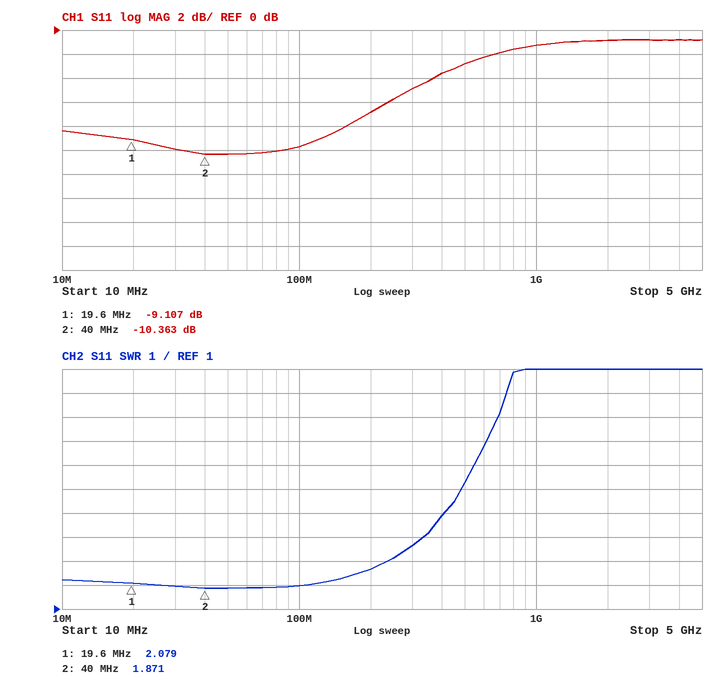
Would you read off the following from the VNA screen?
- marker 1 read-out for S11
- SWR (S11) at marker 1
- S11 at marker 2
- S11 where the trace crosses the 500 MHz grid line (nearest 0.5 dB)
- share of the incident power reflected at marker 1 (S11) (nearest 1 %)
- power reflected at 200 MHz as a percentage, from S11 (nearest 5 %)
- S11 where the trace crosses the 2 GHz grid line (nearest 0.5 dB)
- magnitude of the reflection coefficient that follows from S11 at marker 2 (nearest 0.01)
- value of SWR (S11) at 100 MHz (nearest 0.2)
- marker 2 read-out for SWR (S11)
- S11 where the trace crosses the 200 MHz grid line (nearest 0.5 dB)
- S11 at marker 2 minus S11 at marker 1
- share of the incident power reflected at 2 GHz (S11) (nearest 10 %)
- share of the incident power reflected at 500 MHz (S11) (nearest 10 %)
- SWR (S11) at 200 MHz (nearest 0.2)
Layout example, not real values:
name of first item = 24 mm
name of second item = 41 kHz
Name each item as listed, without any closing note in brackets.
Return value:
marker 1 read-out for S11 = -9.107 dB
SWR (S11) at marker 1 = 2.079
S11 at marker 2 = -10.363 dB
S11 where the trace crosses the 500 MHz grid line = -3.0 dB
share of the incident power reflected at marker 1 (S11) = 12 %
power reflected at 200 MHz as a percentage, from S11 = 20 %
S11 where the trace crosses the 2 GHz grid line = -1.0 dB
magnitude of the reflection coefficient that follows from S11 at marker 2 = 0.30
value of SWR (S11) at 100 MHz = 2.0
marker 2 read-out for SWR = 1.871
S11 where the trace crosses the 200 MHz grid line = -7.0 dB
S11 at marker 2 minus S11 at marker 1 = -1.256 dB
share of the incident power reflected at 2 GHz (S11) = 80 %
share of the incident power reflected at 500 MHz (S11) = 50 %
SWR (S11) at 200 MHz = 2.6
